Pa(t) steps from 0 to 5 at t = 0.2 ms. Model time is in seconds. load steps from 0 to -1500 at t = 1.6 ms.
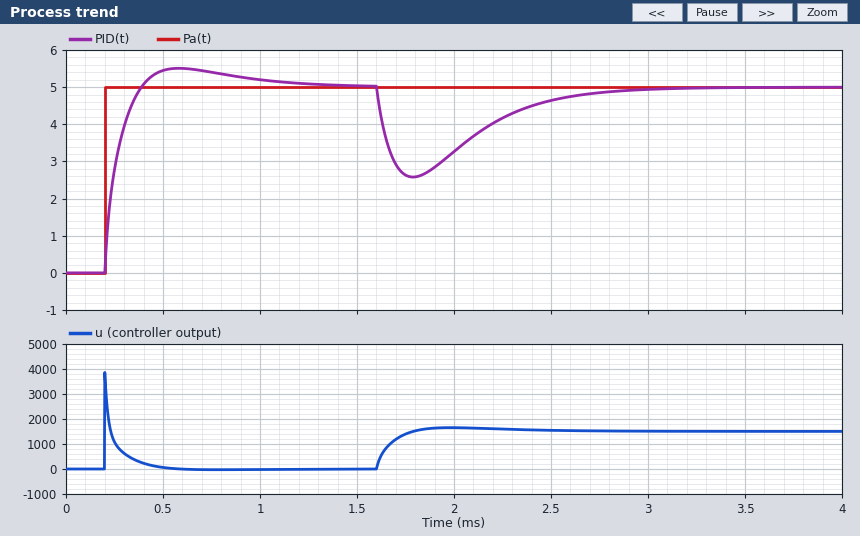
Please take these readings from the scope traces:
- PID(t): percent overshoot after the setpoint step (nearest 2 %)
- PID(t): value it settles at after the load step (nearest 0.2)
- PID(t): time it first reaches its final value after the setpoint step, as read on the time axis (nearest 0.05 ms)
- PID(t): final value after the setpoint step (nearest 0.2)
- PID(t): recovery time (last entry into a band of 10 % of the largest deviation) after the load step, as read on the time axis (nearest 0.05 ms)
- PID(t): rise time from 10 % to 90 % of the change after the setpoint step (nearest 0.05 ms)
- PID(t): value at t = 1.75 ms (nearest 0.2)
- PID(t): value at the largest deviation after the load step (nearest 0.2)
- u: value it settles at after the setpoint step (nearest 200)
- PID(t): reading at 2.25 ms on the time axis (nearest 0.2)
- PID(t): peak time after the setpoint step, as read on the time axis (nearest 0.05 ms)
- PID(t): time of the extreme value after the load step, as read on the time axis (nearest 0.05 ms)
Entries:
10 %
5.0
0.40 ms
5.0
2.60 ms
0.15 ms
2.6
2.6
0
4.2
0.60 ms
1.80 ms
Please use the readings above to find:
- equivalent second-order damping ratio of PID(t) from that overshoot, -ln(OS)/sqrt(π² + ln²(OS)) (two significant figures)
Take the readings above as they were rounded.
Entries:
0.59
